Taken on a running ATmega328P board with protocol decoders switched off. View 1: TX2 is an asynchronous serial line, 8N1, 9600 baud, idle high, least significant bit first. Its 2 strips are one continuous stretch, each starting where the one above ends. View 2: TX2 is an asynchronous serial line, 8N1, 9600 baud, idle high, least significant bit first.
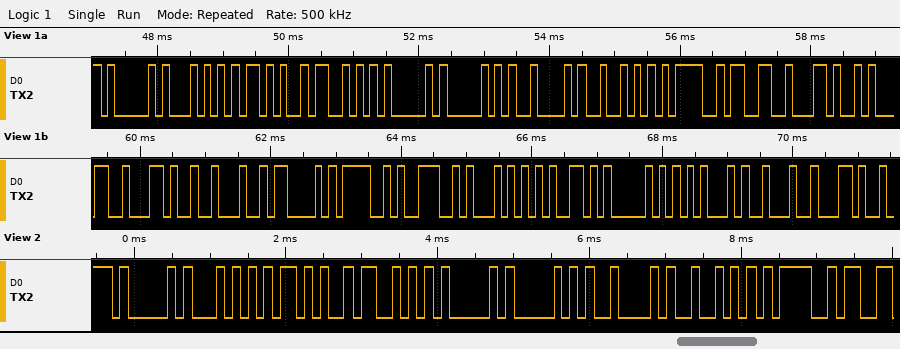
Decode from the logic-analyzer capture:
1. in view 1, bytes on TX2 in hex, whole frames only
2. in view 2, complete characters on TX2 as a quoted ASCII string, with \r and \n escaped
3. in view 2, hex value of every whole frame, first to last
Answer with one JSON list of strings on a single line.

["41 54 2B 53 41 50 42 52 3D 33 2C 31 2C 22 43 4F 4E 54 59 50 45 22 2C", "\"AT+SAPBR=\"", "41 54 2B 53 41 50 42 52 3D"]
